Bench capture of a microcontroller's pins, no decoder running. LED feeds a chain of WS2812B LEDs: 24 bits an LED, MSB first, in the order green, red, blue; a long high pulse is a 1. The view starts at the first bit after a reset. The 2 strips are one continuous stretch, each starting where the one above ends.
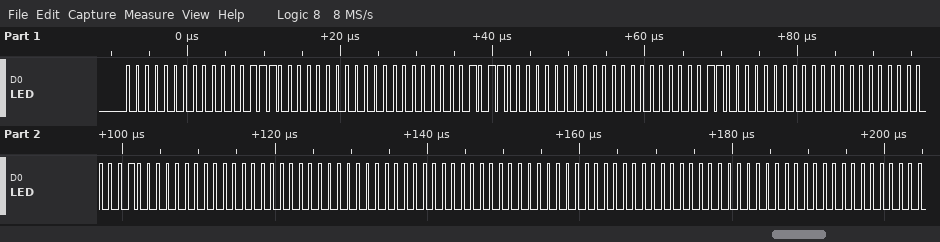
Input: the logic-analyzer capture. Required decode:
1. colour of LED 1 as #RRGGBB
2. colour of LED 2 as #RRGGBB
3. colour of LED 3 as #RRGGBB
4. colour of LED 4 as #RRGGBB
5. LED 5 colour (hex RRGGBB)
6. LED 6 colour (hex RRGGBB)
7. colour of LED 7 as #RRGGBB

#070000
#0B0000
#060000
#010000
#000000
#000000
#000000
